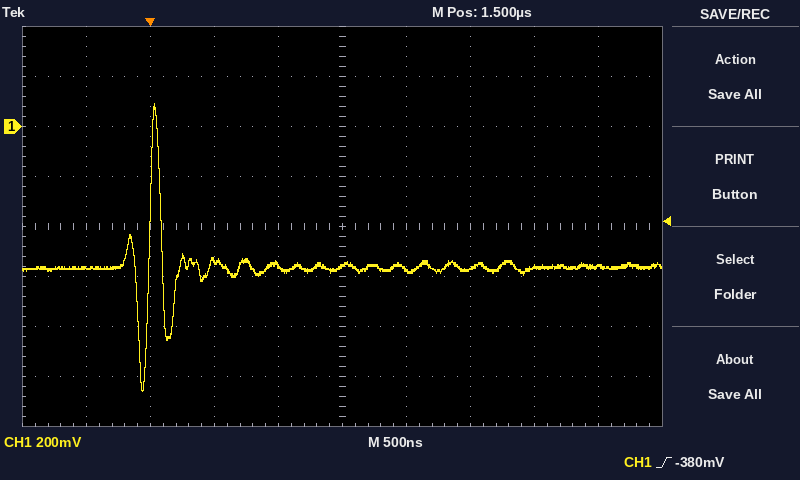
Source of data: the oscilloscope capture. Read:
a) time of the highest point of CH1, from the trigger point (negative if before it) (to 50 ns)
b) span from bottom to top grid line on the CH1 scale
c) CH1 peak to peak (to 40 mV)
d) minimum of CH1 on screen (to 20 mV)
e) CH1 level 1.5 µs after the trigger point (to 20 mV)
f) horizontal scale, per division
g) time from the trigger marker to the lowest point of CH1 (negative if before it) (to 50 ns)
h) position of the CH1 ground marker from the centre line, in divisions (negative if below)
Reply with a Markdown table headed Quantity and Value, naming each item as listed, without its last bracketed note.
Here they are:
| Quantity | Value |
|---|---|
| time of the highest point of CH1, from the trigger point (negative if before it) | +50 ns |
| span from bottom to top grid line on the CH1 scale | 1.6 V |
| CH1 peak to peak | 1.16 V |
| minimum of CH1 on screen | -1.06 V |
| CH1 level 1.5 µs after the trigger point | -560 mV |
| horizontal scale, per division | 500 ns |
| time from the trigger marker to the lowest point of CH1 (negative if before it) | -50 ns |
| position of the CH1 ground marker from the centre line, in divisions | +2.0 div |
